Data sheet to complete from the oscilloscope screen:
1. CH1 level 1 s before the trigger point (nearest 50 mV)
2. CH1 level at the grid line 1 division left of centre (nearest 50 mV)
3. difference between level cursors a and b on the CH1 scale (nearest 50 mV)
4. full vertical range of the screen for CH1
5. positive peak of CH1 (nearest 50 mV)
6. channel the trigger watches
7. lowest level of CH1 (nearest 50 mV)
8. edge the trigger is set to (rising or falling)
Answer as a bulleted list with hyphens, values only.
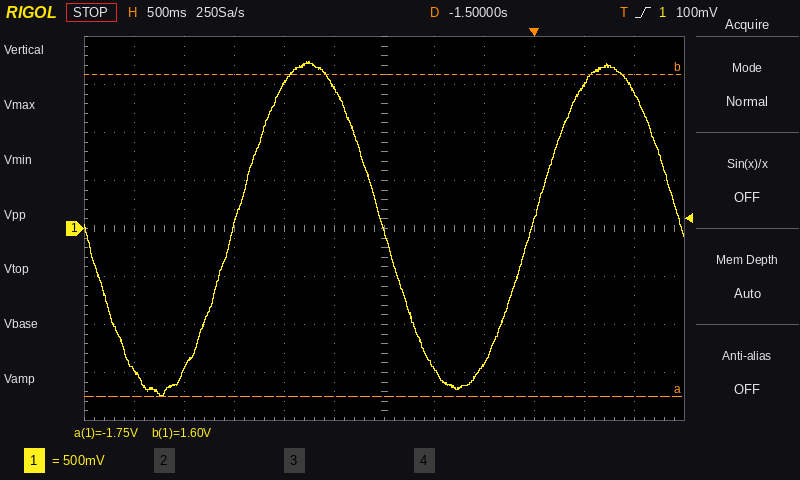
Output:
- -1.45 V
- 1.45 V
- 3.35 V
- 4 V
- 1.75 V
- CH1
- -1.75 V
- rising
